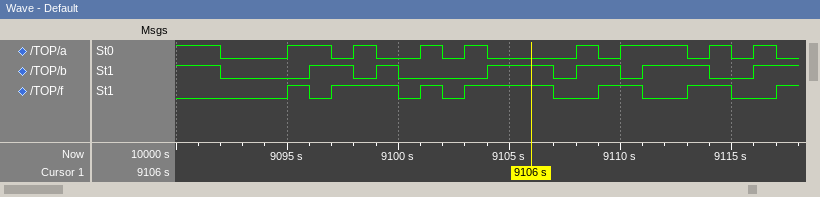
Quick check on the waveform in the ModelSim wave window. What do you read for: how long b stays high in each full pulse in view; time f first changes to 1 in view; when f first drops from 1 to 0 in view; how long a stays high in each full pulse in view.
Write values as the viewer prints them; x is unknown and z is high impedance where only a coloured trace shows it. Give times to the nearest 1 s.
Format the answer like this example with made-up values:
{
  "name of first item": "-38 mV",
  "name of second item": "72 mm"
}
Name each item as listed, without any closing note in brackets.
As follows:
{
  "how long b stays high in each full pulse in view": "2 s, 1 s, 3 s, 2 s, 3 s",
  "time f first changes to 1 in view": "9095 s",
  "when f first drops from 1 to 0 in view": "9096 s",
  "how long a stays high in each full pulse in view": "2 s, 1 s, 1 s, 1 s, 1 s, 3 s, 1 s, 1 s"
}
